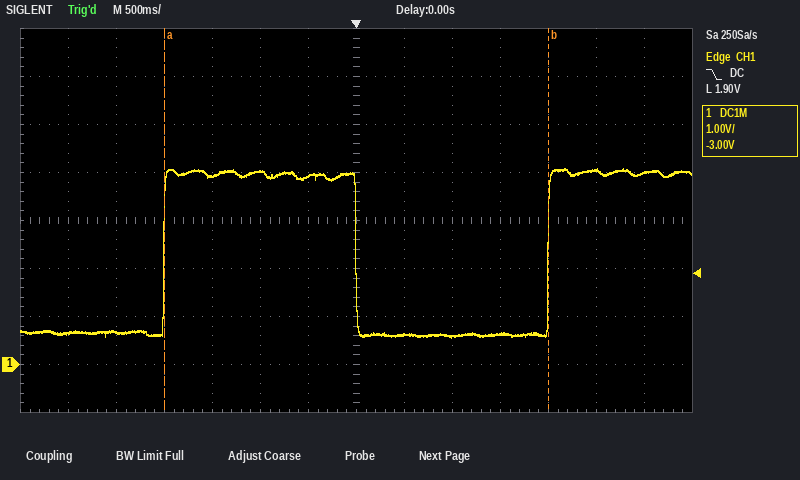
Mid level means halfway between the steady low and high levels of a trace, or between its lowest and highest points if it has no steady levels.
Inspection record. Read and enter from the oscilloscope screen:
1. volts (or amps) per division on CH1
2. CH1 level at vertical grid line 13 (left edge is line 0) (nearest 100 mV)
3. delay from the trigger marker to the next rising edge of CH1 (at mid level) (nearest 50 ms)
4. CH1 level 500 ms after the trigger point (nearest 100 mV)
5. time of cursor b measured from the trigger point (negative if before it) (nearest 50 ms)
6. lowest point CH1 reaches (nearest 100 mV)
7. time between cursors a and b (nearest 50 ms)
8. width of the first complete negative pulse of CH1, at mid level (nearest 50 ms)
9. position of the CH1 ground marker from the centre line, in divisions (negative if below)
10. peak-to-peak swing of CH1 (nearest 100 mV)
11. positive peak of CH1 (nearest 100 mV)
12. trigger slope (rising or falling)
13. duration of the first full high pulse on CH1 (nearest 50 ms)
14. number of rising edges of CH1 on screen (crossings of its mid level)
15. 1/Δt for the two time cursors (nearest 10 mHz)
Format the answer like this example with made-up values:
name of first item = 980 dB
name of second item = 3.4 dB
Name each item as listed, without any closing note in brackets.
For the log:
volts (or amps) per division on CH1 = 1 V
CH1 level at vertical grid line 13 (left edge is line 0) = 4.0 V
delay from the trigger marker to the next rising edge of CH1 (at mid level) = 2.00 s
CH1 level 500 ms after the trigger point = 600 mV
time of cursor b measured from the trigger point (negative if before it) = +2.00 s
lowest point CH1 reaches = 600 mV
time between cursors a and b = 4.00 s
width of the first complete negative pulse of CH1, at mid level = 2.00 s
position of the CH1 ground marker from the centre line, in divisions = -3.0 div
peak-to-peak swing of CH1 = 3.5 V
positive peak of CH1 = 4.1 V
trigger slope = falling
duration of the first full high pulse on CH1 = 2.00 s
number of rising edges of CH1 on screen = 2
1/Δt for the two time cursors = 250 mHz
